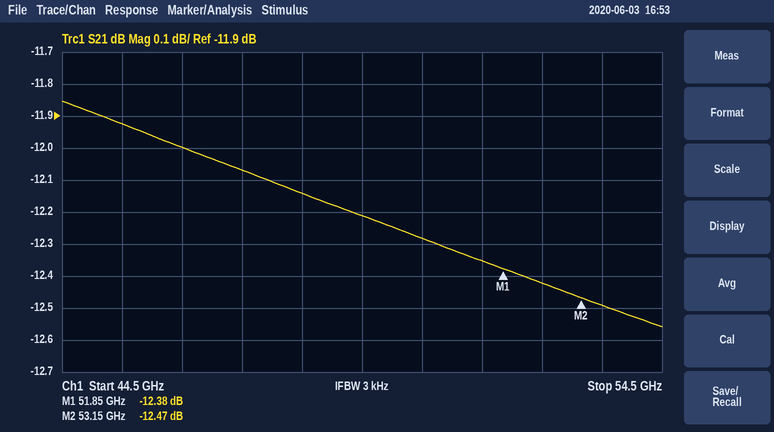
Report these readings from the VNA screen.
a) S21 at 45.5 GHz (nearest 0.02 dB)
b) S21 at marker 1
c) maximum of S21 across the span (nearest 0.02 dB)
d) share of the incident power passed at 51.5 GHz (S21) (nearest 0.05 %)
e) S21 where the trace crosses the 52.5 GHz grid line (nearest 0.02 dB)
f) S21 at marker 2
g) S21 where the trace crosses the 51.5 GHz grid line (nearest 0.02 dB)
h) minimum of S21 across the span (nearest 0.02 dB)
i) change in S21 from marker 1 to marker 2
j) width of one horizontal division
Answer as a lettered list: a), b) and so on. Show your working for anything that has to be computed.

a) -11.92 dB
b) -12.38 dB
c) -11.86 dB
d) 10^(-12.36/10) ≈ 5.81 %, so 5.80 % to the nearest 0.05 %
e) -12.42 dB
f) -12.47 dB
g) -12.36 dB
h) -12.56 dB
i) -12.47 − (-12.38) = -0.09 dB
j) 1 GHz
